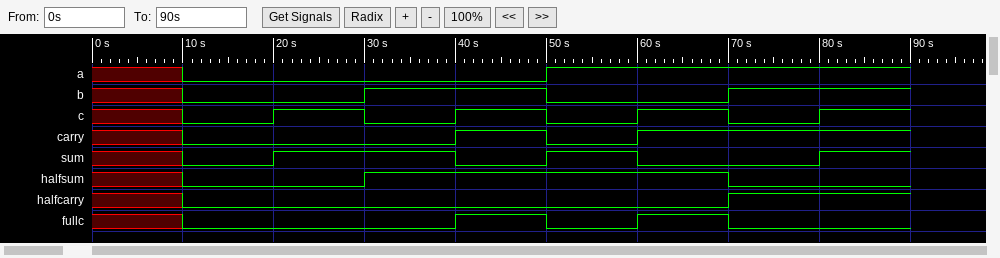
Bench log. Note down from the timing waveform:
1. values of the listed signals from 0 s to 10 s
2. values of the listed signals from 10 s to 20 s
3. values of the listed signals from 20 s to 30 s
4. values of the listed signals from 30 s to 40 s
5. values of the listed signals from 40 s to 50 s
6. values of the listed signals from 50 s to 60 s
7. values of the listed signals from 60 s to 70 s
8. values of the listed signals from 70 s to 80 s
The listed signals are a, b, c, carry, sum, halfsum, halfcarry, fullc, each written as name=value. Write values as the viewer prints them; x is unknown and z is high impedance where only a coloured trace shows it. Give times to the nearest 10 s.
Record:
a=x, b=x, c=x, carry=x, sum=x, halfsum=x, halfcarry=x, fullc=x
a=0, b=0, c=0, carry=0, sum=0, halfsum=0, halfcarry=0, fullc=0
a=0, b=0, c=1, carry=0, sum=1, halfsum=0, halfcarry=0, fullc=0
a=0, b=1, c=0, carry=0, sum=1, halfsum=1, halfcarry=0, fullc=0
a=0, b=1, c=1, carry=1, sum=0, halfsum=1, halfcarry=0, fullc=1
a=1, b=0, c=0, carry=0, sum=1, halfsum=1, halfcarry=0, fullc=0
a=1, b=0, c=1, carry=1, sum=0, halfsum=1, halfcarry=0, fullc=1
a=1, b=1, c=0, carry=1, sum=0, halfsum=0, halfcarry=1, fullc=0
